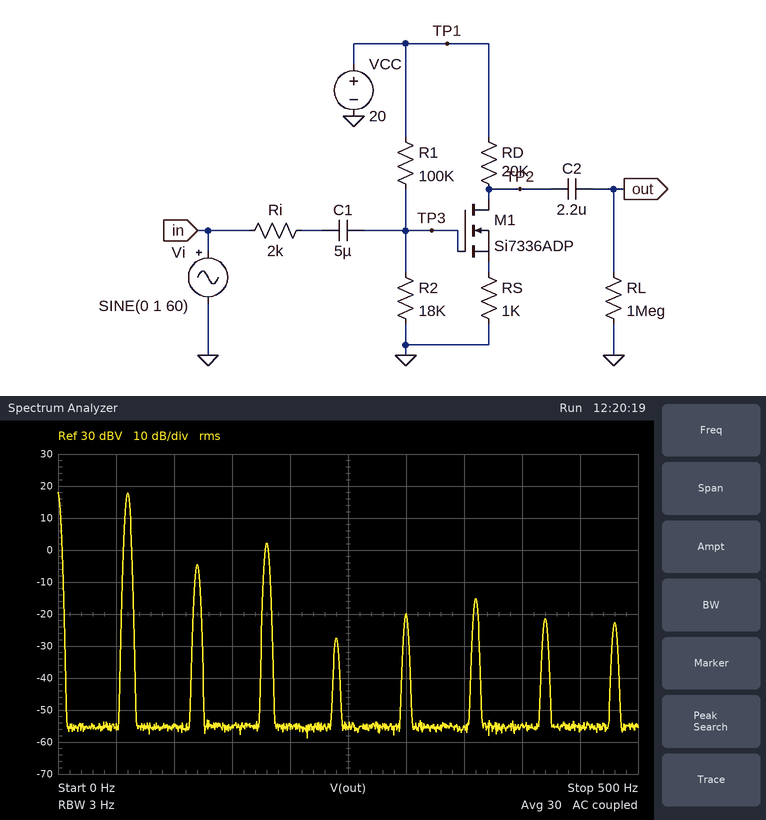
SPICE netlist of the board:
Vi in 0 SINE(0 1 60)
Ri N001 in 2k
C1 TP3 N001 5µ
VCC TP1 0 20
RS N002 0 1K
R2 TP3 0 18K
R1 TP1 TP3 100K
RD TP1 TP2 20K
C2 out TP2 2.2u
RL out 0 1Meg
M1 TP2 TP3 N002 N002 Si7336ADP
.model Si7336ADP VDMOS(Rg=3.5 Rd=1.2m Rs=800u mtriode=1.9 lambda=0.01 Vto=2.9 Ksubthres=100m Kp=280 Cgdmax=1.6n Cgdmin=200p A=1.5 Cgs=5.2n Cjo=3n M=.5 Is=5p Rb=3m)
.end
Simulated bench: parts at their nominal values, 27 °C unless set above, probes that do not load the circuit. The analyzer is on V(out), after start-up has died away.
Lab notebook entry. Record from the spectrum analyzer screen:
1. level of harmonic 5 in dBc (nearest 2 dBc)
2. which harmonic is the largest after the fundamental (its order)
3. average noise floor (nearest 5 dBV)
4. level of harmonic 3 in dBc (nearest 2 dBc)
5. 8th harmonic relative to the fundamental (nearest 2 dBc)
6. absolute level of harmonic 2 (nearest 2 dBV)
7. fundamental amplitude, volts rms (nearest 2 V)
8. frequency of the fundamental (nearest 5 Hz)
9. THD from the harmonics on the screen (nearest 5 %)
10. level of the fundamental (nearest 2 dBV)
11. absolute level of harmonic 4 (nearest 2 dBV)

-38 dBc
3
-55 dBV
-16 dBc
-40 dBc
-4 dBV
8 V
60 Hz
20 %
18 dBV
-28 dBV
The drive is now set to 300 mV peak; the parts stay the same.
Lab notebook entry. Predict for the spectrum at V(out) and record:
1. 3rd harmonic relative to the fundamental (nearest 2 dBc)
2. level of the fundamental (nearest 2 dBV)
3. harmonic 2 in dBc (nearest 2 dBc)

-56 dBc
10 dBV
-40 dBc
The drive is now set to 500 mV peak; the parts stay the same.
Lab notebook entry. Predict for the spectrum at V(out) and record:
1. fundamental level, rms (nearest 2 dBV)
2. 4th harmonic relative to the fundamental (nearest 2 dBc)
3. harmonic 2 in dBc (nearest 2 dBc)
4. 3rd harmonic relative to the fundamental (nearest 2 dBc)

14 dBV
-52 dBc
-34 dBc
-44 dBc
